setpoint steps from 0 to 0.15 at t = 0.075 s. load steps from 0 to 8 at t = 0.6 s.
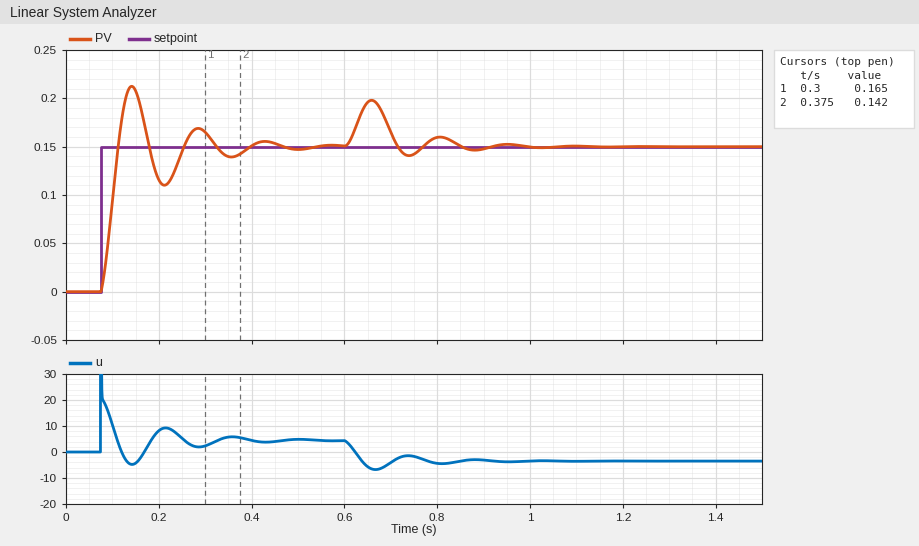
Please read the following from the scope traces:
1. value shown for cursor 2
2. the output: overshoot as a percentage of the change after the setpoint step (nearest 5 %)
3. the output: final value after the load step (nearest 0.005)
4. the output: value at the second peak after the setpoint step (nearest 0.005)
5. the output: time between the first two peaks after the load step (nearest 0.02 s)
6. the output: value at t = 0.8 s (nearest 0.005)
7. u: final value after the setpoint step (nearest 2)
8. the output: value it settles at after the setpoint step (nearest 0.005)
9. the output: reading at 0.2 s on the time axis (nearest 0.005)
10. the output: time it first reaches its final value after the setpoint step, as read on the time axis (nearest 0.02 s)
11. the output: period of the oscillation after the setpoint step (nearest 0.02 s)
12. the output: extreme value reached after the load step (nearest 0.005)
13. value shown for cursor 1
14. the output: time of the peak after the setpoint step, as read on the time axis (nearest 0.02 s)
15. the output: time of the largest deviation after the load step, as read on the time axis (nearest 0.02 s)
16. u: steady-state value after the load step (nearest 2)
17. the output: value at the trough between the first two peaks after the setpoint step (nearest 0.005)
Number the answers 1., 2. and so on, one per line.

1. 0.142
2. 40 %
3. 0.150
4. 0.170
5. 0.14 s
6. 0.160
7. 4
8. 0.150
9. 0.115
10. 0.12 s
11. 0.14 s
12. 0.200
13. 0.165
14. 0.14 s
15. 0.66 s
16. -4
17. 0.110
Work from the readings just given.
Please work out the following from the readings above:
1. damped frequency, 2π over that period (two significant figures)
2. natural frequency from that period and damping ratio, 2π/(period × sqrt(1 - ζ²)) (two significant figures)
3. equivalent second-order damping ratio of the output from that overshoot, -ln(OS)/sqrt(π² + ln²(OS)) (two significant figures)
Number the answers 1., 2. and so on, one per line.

1. 45 rad/s
2. 47 rad/s
3. 0.28
